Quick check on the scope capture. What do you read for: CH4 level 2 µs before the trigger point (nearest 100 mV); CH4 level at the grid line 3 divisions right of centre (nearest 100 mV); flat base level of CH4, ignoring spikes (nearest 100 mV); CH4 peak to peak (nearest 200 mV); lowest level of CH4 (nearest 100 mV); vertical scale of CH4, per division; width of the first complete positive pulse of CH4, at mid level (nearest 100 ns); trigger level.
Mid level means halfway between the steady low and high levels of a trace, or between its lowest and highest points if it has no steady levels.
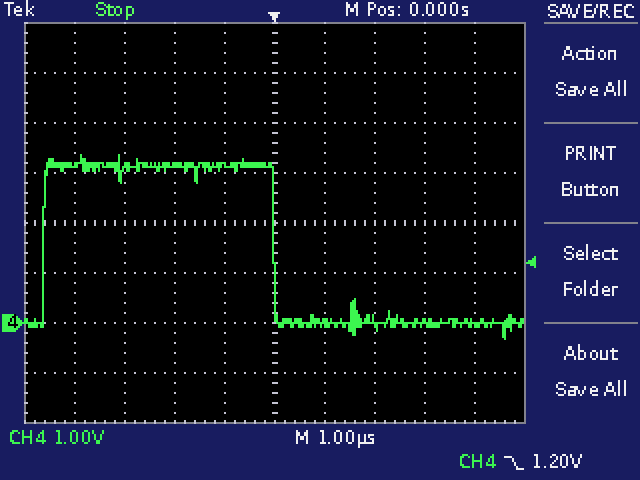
3.2 V
0.0 V
0.0 V
3.6 V
-300 mV
1 V
4.6 µs
1.20 V
